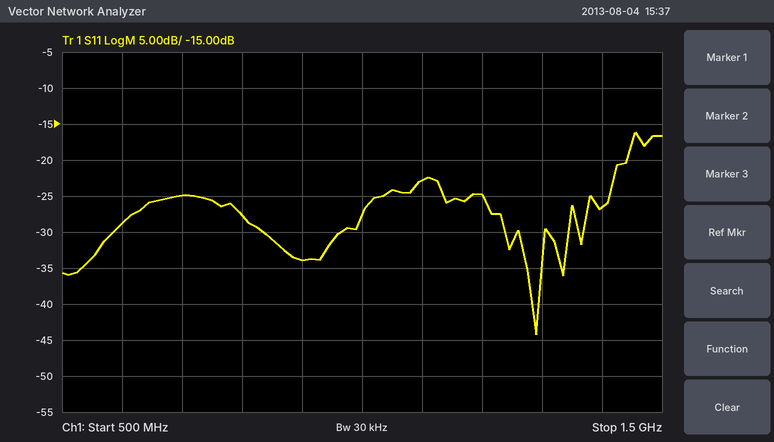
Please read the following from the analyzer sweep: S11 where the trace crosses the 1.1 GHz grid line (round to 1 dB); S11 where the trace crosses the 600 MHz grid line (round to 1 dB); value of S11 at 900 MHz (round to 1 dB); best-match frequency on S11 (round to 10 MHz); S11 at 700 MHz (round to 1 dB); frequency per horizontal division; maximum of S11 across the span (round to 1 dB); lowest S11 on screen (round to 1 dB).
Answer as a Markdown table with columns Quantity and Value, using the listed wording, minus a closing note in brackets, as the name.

| Quantity | Value |
|---|---|
| S11 where the trace crosses the 1.1 GHz grid line | -23 dB |
| S11 where the trace crosses the 600 MHz grid line | -29 dB |
| value of S11 at 900 MHz | -34 dB |
| best-match frequency on S11 | 1.29 GHz |
| S11 at 700 MHz | -25 dB |
| frequency per horizontal division | 100 MHz |
| maximum of S11 across the span | -16 dB |
| lowest S11 on screen | -44 dB |
